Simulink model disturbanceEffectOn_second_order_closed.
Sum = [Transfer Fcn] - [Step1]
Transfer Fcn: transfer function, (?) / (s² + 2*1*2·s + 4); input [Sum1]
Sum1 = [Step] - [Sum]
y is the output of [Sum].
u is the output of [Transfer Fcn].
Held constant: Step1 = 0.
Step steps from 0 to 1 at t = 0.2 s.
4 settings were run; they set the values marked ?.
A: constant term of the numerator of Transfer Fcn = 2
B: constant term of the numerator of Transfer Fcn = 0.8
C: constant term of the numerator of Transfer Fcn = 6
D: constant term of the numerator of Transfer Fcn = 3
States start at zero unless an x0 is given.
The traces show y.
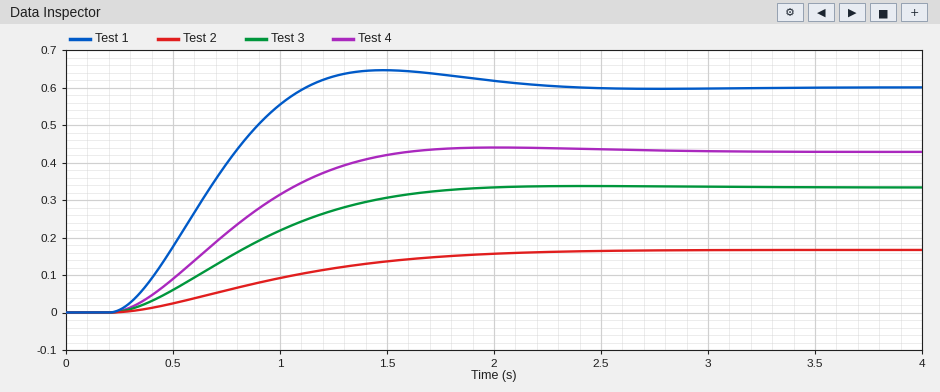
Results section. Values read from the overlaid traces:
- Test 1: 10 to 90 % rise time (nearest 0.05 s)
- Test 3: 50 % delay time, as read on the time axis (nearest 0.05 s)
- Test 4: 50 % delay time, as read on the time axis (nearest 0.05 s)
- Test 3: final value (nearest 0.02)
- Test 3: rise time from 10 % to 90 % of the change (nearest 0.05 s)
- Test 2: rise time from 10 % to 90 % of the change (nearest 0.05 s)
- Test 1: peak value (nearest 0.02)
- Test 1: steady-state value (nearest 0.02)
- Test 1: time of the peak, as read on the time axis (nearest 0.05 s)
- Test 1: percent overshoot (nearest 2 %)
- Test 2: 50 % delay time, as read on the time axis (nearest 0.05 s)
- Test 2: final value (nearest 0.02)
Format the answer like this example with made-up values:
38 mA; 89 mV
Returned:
0.60 s; 0.80 s; 0.75 s; 0.34; 1.05 s; 1.35 s; 0.64; 0.60; 1.50 s; 8 %; 0.95 s; 0.16
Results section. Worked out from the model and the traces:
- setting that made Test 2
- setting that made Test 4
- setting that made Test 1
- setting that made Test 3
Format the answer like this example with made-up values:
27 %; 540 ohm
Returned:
B; D; C; A
